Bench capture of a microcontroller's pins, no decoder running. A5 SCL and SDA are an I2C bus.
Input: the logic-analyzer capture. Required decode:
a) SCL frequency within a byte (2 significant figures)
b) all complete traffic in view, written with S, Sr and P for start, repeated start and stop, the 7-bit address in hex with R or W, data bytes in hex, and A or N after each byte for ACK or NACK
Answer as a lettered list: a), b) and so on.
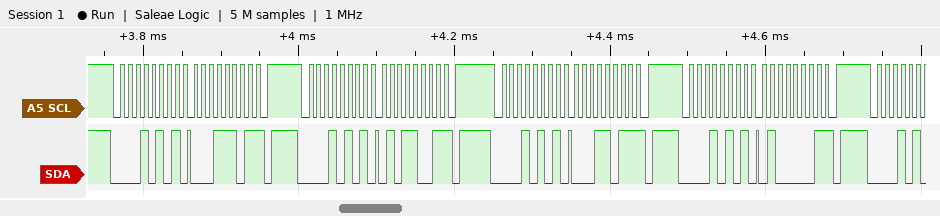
a) 100 kHz
b) S 0AR A 1D N P S 0AR A 59 N P S 0AR A 1B N P S 0AR A 41 N P
